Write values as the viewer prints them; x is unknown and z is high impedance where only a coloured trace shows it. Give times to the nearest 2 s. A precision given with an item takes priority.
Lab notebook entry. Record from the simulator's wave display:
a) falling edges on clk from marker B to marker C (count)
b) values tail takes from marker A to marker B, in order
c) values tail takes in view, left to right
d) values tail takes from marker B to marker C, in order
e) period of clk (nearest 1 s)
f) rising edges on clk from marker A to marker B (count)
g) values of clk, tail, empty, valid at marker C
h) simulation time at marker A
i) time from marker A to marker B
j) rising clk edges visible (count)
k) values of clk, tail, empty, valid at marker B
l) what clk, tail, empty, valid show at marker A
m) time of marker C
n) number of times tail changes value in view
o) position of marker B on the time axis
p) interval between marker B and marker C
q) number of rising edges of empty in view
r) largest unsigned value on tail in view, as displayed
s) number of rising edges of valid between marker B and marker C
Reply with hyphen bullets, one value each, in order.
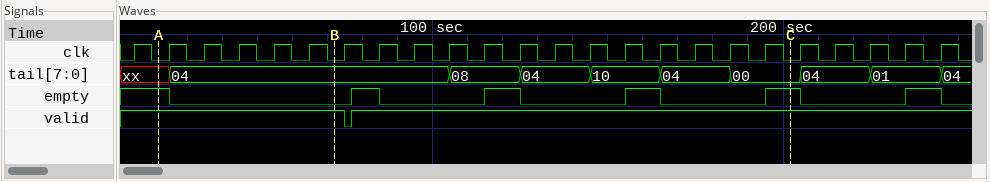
- 13
- xx, 04
- xx, 04, 08, 04, 10, 04, 00, 04, 01, 04
- 04, 08, 04, 10, 04, 00
- 10 s
- 5
- clk=0, tail=00, empty=1, valid=1
- 22 s
- 50 s
- 24
- clk=0, tail=04, empty=0, valid=1
- clk=0, tail=xx, empty=1, valid=1
- 202 s
- 9
- 72 s
- 130 s
- 5
- 10
- 1
